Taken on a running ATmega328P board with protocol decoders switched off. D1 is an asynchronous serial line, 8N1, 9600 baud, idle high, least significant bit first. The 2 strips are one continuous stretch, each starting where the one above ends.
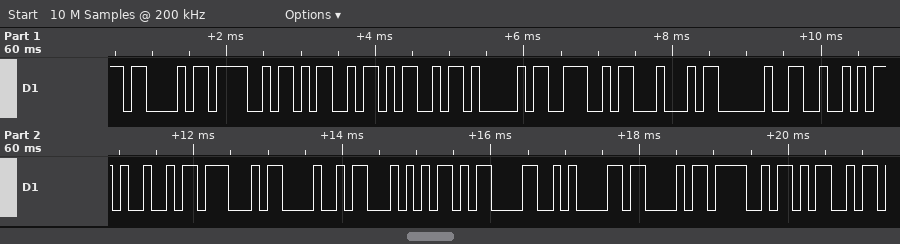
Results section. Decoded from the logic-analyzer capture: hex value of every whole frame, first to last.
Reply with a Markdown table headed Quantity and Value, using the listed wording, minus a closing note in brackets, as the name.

| Quantity | Value |
|---|---|
| hex value of every whole frame, first to last | 0x43 0x4F 0x4D 0x4D 0x41 0x4E 0x44 0x20 0x52 0x49 0x47 0x48 0x54 0x0D 0x0A 0x43 0x4F 0x4D |
